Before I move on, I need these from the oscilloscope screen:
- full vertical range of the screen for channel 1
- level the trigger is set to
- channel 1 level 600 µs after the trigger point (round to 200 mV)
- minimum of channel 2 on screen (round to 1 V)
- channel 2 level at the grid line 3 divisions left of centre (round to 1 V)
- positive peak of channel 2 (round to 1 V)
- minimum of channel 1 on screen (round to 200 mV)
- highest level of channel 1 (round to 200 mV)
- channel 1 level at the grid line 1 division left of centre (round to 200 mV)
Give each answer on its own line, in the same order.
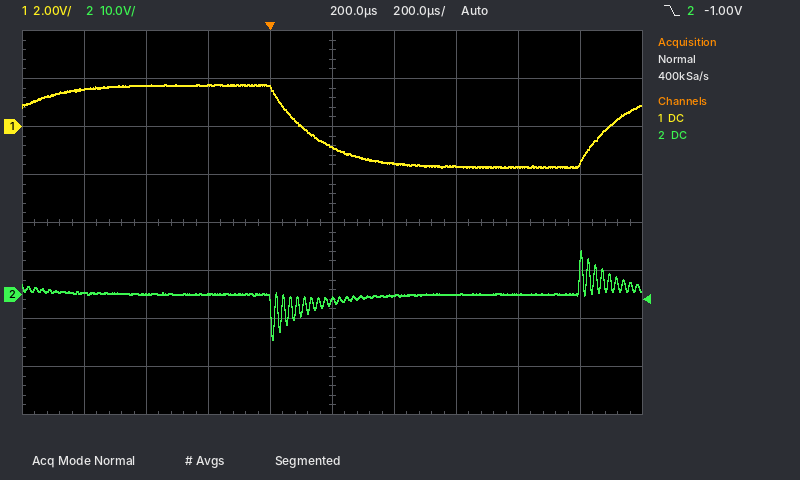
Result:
16 V
-1.00 V
-1.6 V
-9 V
0 V
9 V
-1.8 V
1.8 V
1.6 V
